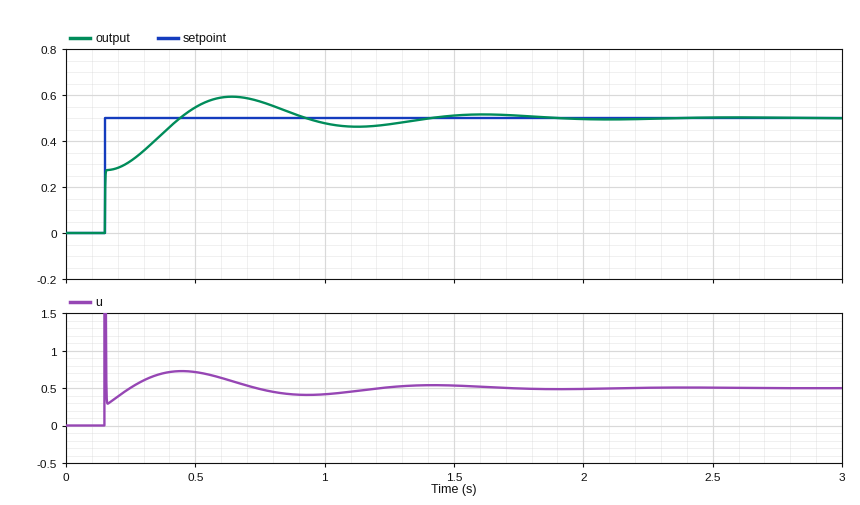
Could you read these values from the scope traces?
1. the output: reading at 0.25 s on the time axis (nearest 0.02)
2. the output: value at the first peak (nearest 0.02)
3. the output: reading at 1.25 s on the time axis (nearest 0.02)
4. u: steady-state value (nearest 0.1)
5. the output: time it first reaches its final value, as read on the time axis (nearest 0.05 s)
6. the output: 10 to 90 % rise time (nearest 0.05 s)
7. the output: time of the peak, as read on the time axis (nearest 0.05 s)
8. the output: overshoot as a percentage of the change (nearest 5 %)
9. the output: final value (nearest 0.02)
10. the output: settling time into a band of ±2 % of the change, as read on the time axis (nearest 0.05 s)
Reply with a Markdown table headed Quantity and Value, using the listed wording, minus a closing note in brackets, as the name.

| Quantity | Value |
|---|---|
| the output: reading at 0.25 s on the time axis | 0.32 |
| the output: value at the first peak | 0.60 |
| the output: reading at 1.25 s on the time axis | 0.48 |
| u: steady-state value | 0.5 |
| the output: time it first reaches its final value, as read on the time axis | 0.45 s |
| the output: 10 to 90 % rise time | 0.25 s |
| the output: time of the peak, as read on the time axis | 0.65 s |
| the output: overshoot as a percentage of the change | 20 % |
| the output: final value | 0.50 |
| the output: settling time into a band of ±2 % of the change, as read on the time axis | 1.75 s |
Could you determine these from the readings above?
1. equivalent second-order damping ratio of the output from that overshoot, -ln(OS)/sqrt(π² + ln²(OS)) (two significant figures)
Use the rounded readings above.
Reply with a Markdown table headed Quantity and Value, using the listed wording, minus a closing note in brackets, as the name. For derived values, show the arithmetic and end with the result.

| Quantity | Value |
|---|---|
| equivalent second-order damping ratio of the output from that overshoot, -ln(OS)/sqrt(π² + ln²(OS)) | ln(0.2) = -1.609; 1.609 / sqrt(9.870 + 2.590) = 0.46 |
